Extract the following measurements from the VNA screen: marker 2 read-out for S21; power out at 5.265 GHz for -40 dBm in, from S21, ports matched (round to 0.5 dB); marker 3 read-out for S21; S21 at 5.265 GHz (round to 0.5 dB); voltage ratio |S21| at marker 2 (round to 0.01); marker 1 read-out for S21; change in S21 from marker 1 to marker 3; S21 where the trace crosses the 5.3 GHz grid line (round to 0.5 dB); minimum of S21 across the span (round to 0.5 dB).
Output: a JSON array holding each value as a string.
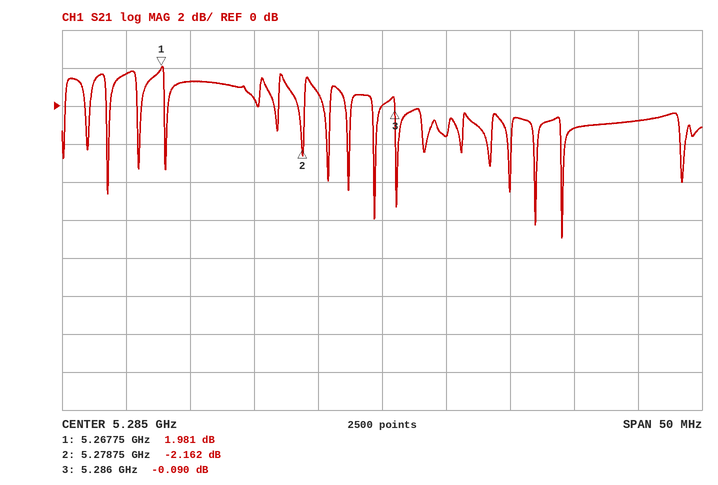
["-2.162 dB", "-38.5 dBm", "-0.090 dB", "1.5 dB", "0.78", "1.981 dB", "-2.071 dB", "-1.0 dB", "-7.0 dB"]
